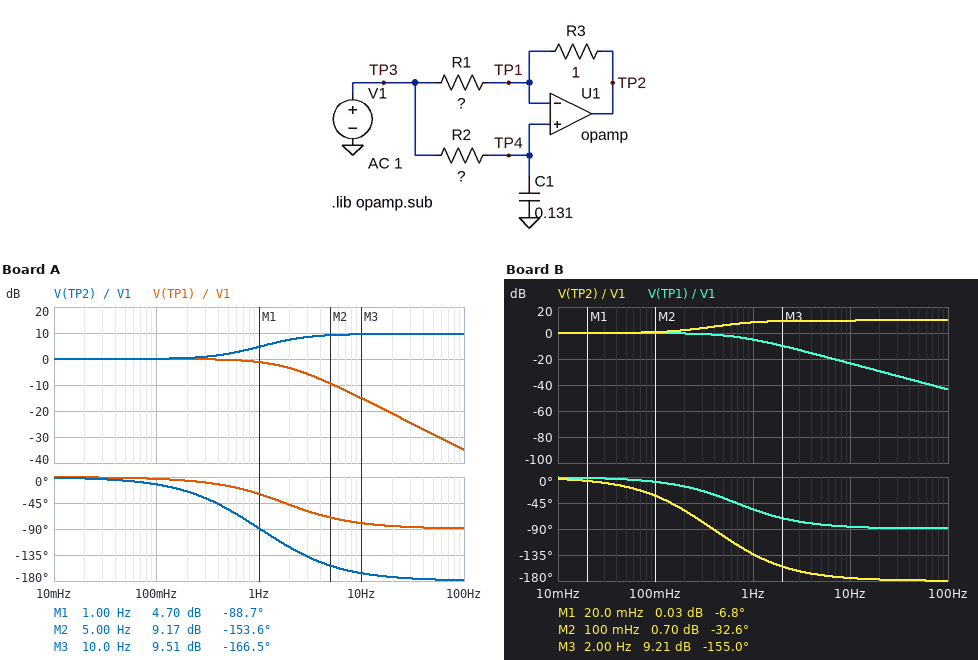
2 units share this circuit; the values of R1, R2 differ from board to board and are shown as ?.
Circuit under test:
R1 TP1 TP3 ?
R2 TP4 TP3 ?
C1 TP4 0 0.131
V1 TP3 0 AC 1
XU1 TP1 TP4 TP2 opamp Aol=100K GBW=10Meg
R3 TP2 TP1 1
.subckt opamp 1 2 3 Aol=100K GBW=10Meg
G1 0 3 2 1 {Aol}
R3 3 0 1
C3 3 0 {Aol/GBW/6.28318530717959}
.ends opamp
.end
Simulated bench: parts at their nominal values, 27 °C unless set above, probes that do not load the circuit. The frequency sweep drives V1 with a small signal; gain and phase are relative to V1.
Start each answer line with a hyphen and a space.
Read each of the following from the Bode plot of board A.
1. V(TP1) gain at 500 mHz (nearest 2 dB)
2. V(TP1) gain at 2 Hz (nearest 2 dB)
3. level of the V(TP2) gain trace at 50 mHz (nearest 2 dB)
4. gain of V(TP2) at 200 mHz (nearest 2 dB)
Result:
- 0 dB
- -4 dB
- 0 dB
- 0 dB
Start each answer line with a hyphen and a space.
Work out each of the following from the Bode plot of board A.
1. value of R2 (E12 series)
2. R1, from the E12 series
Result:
- 0.68 Ω
- 0.33 Ω
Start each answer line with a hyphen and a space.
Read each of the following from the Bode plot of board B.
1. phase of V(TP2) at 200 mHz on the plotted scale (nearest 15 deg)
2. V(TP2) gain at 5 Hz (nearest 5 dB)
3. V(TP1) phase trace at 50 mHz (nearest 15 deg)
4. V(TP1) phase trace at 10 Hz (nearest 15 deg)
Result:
- -60 deg
- 10 dB
- 0 deg
- -90 deg
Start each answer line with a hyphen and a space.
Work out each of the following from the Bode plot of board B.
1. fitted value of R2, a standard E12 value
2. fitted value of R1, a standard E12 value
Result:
- 1.8 Ω
- 0.33 Ω
